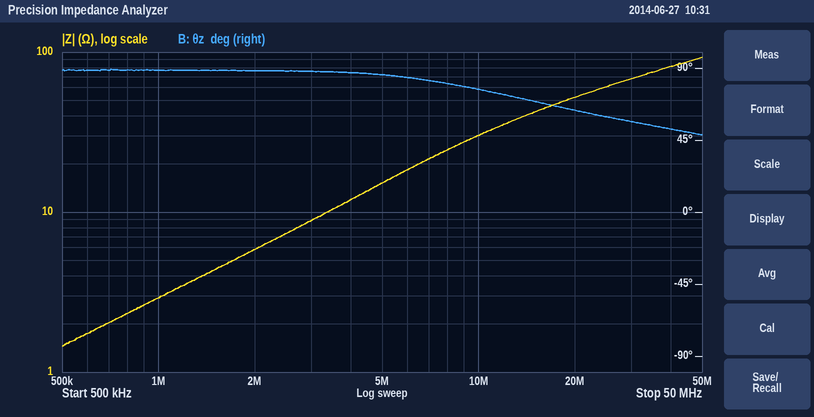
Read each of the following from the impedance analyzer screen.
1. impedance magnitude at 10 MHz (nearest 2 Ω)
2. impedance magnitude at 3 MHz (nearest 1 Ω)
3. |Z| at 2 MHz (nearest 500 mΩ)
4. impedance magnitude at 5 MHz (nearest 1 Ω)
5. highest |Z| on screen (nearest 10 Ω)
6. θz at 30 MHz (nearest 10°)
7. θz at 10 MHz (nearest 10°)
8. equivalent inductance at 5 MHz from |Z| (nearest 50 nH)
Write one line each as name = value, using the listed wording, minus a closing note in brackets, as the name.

impedance magnitude at 10 MHz = 30 Ω
impedance magnitude at 3 MHz = 9 Ω
|Z| at 2 MHz = 6.0 Ω
impedance magnitude at 5 MHz = 15 Ω
highest |Z| on screen = 90 Ω
θz at 30 MHz = 60°
θz at 10 MHz = 80°
equivalent inductance at 5 MHz from |Z| = 500 nH
